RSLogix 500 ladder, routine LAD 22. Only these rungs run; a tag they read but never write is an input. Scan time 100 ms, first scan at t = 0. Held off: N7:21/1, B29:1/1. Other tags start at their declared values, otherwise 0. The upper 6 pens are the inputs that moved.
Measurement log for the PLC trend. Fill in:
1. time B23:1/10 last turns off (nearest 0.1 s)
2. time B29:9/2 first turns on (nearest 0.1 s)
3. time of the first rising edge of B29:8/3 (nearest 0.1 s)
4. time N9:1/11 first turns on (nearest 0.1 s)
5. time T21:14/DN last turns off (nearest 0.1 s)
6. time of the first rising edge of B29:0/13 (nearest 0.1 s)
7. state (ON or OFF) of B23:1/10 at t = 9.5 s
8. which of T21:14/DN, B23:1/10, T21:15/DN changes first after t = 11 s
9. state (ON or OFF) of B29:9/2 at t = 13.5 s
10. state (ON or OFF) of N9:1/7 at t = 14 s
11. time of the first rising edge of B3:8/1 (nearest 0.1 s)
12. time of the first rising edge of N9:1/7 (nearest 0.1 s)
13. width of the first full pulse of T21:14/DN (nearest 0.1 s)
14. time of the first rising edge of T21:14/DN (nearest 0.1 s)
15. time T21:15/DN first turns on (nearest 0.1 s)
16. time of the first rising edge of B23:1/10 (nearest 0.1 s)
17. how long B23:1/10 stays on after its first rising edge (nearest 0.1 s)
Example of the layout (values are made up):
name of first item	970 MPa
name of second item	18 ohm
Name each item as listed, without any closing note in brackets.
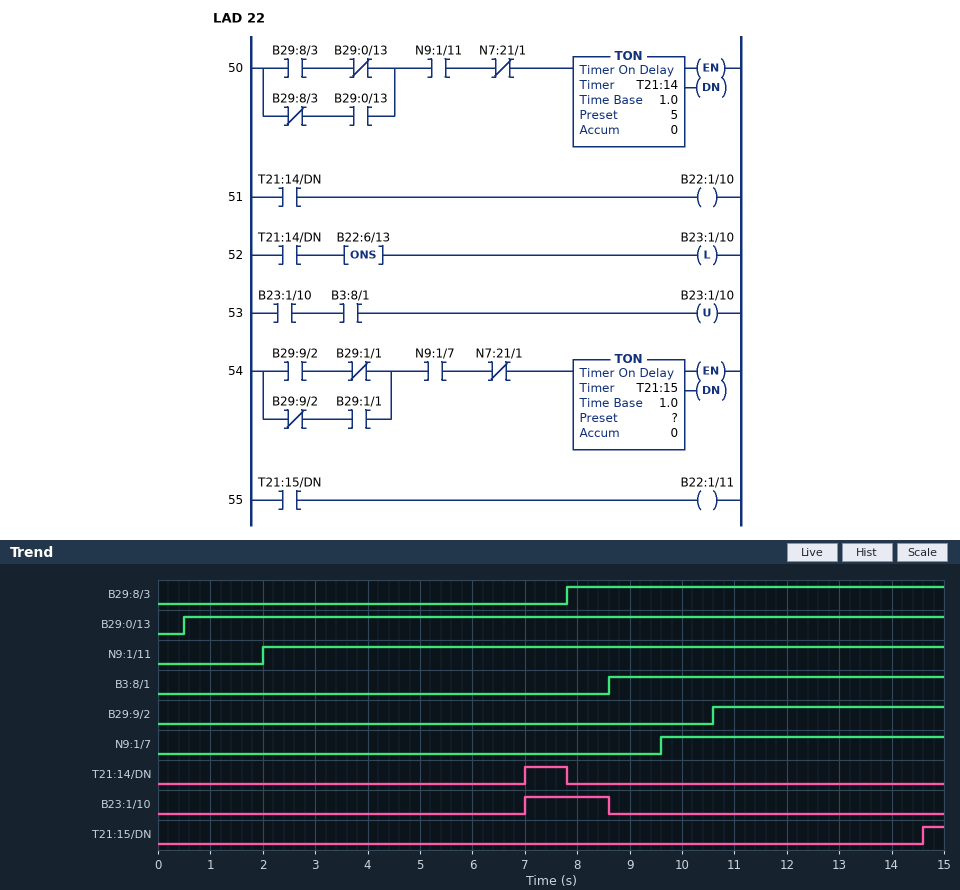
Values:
time B23:1/10 last turns off	8.6 s
time B29:9/2 first turns on	10.6 s
time of the first rising edge of B29:8/3	7.8 s
time N9:1/11 first turns on	2.0 s
time T21:14/DN last turns off	7.8 s
time of the first rising edge of B29:0/13	0.5 s
state (ON or OFF) of B23:1/10 at t = 9.5 s	OFF
which of T21:14/DN, B23:1/10, T21:15/DN changes first after t = 11 s	T21:15/DN
state (ON or OFF) of B29:9/2 at t = 13.5 s	ON
state (ON or OFF) of N9:1/7 at t = 14 s	ON
time of the first rising edge of B3:8/1	8.6 s
time of the first rising edge of N9:1/7	9.6 s
width of the first full pulse of T21:14/DN	0.8 s
time of the first rising edge of T21:14/DN	7.0 s
time T21:15/DN first turns on	14.6 s
time of the first rising edge of B23:1/10	7.0 s
how long B23:1/10 stays on after its first rising edge	1.6 s
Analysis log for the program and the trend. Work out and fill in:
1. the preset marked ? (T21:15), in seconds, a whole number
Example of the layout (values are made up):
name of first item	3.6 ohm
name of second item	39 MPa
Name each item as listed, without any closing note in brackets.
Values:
the preset marked ? (T21:15), in seconds, a whole number	4 s
